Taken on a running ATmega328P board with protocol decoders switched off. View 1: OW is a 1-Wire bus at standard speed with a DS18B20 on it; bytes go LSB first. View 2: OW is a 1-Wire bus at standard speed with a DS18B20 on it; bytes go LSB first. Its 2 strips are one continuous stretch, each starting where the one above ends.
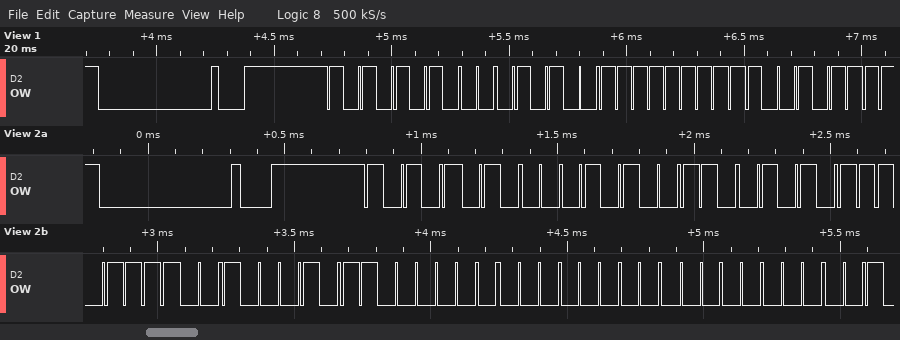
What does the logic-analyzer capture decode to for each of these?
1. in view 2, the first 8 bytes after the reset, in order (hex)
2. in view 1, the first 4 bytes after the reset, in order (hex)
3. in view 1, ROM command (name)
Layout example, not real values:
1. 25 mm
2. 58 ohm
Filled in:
1. 55 28 53 F7 44 03 00 00
2. 55 28 FF D3
3. Match ROM
